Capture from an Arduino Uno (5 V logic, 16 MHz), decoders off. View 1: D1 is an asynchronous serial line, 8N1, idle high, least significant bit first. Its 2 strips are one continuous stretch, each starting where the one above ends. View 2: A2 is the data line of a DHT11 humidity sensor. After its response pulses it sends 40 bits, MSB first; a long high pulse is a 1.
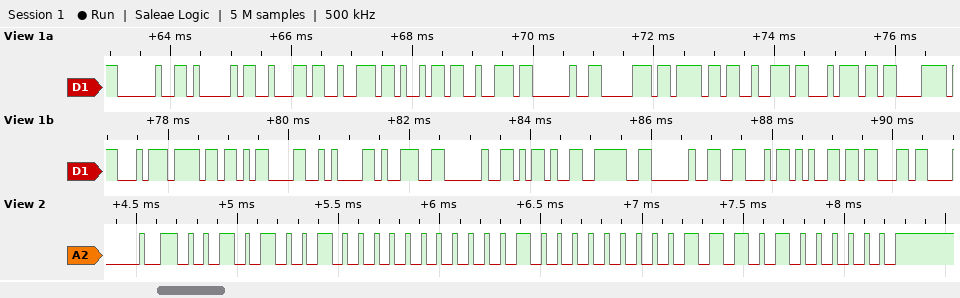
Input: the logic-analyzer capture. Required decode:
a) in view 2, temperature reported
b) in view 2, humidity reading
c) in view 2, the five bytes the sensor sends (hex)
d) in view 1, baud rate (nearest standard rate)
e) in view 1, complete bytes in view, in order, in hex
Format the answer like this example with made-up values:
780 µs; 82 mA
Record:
16.7 °C; 41 %; 29 00 10 07 40; 9600 baud; 20 41 62 72 69 72 20 70 6F 72 74 C3 A3 6F 0D 0A 39 20 2D 3E 20 46 65 63
